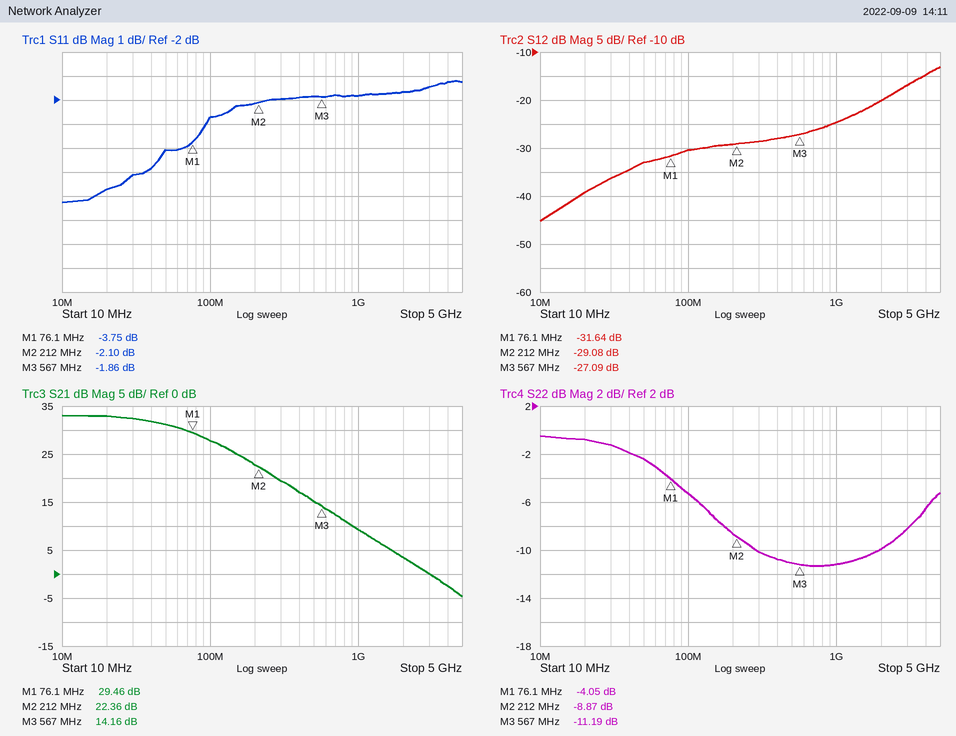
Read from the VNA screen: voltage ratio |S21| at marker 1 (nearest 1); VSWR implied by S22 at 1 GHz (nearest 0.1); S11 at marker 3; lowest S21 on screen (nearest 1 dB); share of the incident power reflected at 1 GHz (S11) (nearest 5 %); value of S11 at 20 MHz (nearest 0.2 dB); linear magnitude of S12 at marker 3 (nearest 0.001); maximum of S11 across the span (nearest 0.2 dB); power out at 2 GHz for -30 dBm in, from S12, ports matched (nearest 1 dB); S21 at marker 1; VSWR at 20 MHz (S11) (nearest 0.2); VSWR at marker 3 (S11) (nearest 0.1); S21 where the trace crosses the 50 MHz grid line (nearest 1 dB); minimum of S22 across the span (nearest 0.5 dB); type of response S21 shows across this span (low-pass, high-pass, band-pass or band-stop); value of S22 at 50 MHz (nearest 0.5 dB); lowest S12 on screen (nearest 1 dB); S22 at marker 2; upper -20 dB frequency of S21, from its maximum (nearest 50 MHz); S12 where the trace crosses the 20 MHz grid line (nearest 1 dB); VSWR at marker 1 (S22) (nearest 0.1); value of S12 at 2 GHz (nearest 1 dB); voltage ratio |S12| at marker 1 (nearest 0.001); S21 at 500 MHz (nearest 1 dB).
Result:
30
1.8
-1.86 dB
-5 dB
65 %
-5.8 dB
0.044
-1.2 dB
-50 dBm
29.46 dB
3.2
9.4
31 dB
-11.5 dB
low-pass
-2.5 dB
-45 dB
-8.87 dB
650 MHz
-39 dB
4.4
-20 dB
0.026
15 dB
